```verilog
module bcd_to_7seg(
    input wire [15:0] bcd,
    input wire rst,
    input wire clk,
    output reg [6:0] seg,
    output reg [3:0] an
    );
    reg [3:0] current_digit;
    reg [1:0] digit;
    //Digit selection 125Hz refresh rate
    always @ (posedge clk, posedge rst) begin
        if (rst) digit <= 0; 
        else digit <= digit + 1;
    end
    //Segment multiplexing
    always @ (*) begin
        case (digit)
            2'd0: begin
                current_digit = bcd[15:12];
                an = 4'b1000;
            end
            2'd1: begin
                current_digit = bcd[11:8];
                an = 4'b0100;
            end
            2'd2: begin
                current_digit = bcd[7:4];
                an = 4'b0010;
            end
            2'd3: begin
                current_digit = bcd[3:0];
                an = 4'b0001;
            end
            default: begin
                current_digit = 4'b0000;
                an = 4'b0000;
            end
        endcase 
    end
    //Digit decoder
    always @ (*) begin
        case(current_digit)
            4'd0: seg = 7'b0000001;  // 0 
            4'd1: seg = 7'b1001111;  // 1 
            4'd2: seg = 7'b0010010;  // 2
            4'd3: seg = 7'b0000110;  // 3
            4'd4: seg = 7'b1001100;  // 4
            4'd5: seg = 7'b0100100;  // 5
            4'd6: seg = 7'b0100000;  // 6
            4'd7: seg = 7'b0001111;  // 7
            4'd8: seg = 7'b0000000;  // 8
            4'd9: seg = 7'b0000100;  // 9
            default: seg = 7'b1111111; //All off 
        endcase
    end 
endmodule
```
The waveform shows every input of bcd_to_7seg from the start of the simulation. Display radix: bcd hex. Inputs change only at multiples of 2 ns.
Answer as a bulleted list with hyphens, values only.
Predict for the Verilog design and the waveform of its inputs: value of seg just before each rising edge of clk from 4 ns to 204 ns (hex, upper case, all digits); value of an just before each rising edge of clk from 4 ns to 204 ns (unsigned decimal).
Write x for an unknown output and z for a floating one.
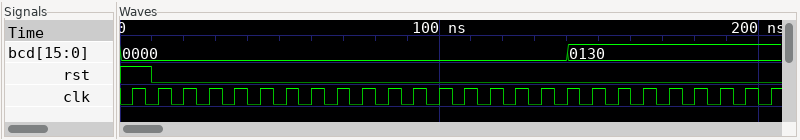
- 01, 01, 01, 01, 01, 01, 01, 01, 01, 01, 01, 01, 01, 01, 01, 01, 01, 01, 4F, 06, 01, 01, 4F, 06, 01, 01
- 8, 8, 4, 2, 1, 8, 4, 2, 1, 8, 4, 2, 1, 8, 4, 2, 1, 8, 4, 2, 1, 8, 4, 2, 1, 8
